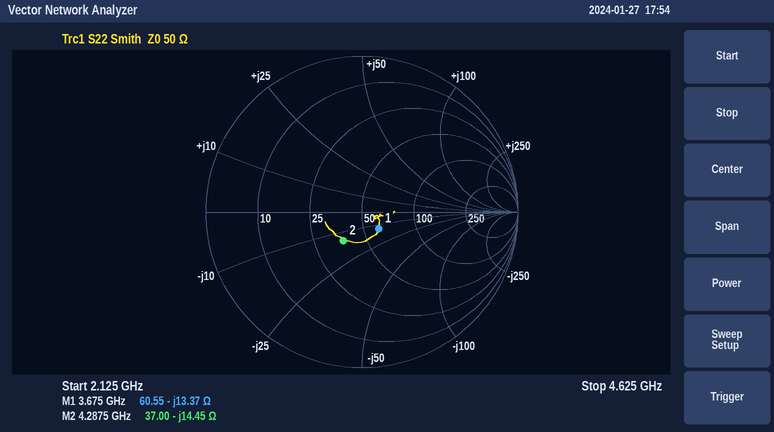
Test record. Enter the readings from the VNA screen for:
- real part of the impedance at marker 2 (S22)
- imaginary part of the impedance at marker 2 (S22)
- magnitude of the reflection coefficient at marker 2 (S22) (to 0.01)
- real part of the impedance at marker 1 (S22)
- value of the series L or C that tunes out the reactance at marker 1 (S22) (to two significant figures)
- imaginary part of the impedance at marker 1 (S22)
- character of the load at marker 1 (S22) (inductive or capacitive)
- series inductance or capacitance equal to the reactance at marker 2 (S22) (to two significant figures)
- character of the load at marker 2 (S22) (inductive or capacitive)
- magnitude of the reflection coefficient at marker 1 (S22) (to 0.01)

37.00 Ω
-14.45 Ω
0.22
60.55 Ω
580 pH
-13.37 Ω
capacitive
2.6 pF
capacitive
0.15
